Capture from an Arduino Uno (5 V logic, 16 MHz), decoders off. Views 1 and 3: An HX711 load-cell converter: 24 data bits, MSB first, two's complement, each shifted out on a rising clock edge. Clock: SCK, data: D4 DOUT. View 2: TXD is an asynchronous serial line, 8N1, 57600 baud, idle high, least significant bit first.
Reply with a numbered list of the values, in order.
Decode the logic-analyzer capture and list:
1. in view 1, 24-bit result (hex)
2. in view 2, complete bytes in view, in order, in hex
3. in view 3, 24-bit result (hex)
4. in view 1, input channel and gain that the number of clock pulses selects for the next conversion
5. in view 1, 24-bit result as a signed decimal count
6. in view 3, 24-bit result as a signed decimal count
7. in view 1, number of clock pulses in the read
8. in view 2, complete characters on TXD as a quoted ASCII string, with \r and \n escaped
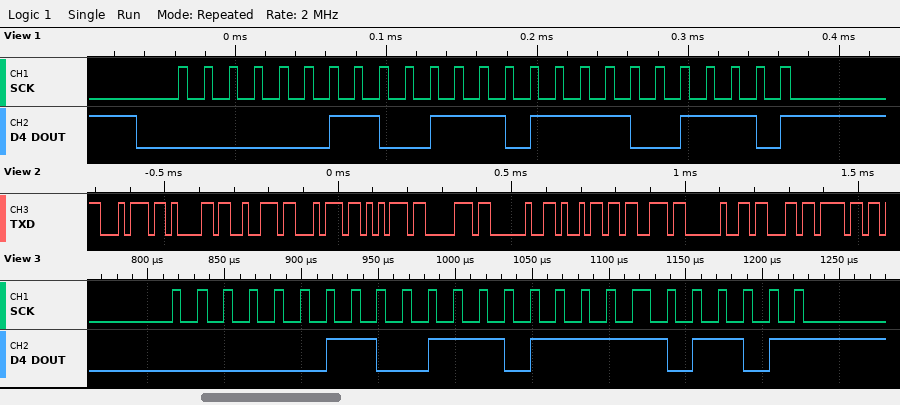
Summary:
1. 0x033BCE
2. 74 61 72 74 75 70 20 69 73 20 63 6F
3. 0x033BED
4. channel A, gain 128
5. 211918
6. 211949
7. 25
8. "tartup is co"
